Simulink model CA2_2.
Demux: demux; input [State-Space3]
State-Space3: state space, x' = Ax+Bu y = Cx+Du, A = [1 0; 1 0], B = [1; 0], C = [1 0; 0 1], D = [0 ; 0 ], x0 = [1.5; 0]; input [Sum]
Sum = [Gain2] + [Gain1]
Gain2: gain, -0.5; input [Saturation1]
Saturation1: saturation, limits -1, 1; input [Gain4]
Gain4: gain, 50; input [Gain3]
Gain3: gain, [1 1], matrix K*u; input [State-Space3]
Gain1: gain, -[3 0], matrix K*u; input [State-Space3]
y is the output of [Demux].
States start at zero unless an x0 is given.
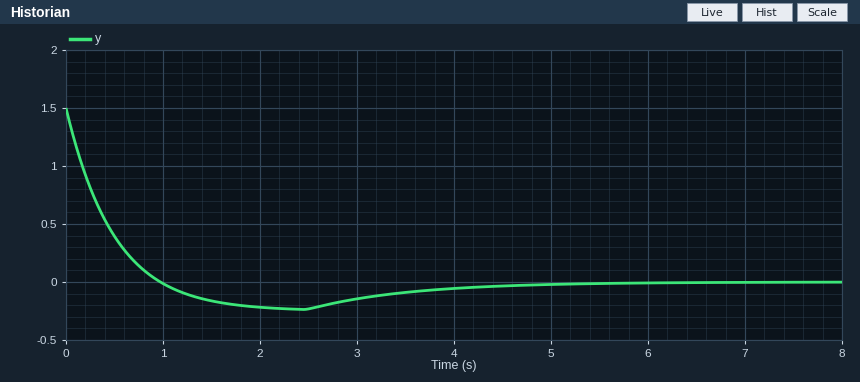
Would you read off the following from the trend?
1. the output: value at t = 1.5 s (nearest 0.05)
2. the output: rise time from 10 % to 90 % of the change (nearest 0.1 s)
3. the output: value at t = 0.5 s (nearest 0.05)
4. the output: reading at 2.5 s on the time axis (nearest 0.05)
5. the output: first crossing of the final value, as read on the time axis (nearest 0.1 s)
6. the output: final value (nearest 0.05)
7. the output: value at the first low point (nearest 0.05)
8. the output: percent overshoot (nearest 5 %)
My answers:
-0.15
0.7 s
0.40
-0.25
1.0 s
0.00
-0.25
15 %
